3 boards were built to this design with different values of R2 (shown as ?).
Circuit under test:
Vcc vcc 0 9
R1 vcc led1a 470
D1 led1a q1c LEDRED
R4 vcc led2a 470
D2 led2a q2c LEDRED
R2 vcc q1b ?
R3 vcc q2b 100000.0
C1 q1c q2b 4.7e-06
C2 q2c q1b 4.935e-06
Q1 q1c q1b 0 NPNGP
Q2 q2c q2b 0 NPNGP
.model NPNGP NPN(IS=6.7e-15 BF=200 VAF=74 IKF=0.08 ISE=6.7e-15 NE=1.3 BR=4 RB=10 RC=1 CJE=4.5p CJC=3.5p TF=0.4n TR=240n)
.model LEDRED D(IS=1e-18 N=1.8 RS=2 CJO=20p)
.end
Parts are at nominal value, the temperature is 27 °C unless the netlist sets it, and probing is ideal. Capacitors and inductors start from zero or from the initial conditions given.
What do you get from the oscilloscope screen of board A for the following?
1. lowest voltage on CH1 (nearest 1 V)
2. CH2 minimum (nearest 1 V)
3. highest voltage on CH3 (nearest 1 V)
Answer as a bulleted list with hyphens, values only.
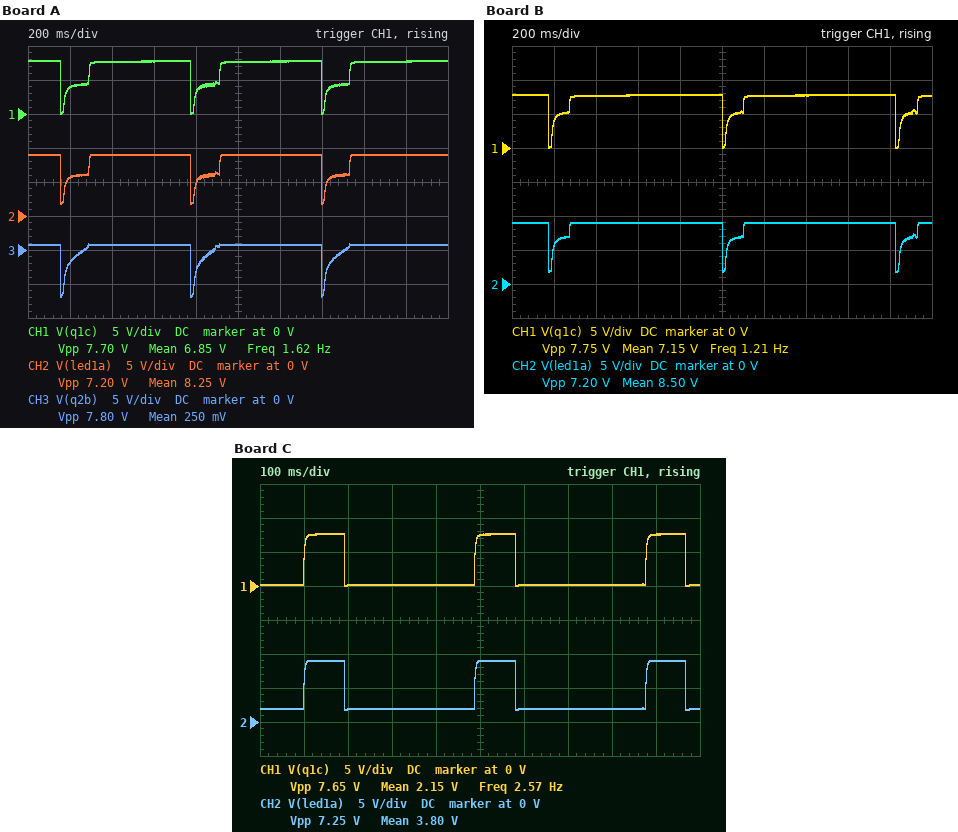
- 0 V
- 2 V
- 1 V
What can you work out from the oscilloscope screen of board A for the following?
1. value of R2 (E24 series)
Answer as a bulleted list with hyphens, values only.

- 200 kΩ
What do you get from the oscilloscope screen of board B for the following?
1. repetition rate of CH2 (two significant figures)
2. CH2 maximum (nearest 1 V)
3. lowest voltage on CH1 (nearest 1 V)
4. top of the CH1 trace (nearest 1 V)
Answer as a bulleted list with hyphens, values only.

- 1.2 Hz
- 9 V
- 0 V
- 8 V
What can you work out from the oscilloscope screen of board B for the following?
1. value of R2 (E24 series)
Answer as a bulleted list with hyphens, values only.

- 300 kΩ
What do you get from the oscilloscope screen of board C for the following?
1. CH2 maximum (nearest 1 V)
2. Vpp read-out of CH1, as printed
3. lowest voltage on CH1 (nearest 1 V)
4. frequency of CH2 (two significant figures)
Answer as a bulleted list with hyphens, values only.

- 9 V
- 7.65 V
- 0 V
- 2.6 Hz
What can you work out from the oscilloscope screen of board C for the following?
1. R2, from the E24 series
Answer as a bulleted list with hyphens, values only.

- 39 kΩ
